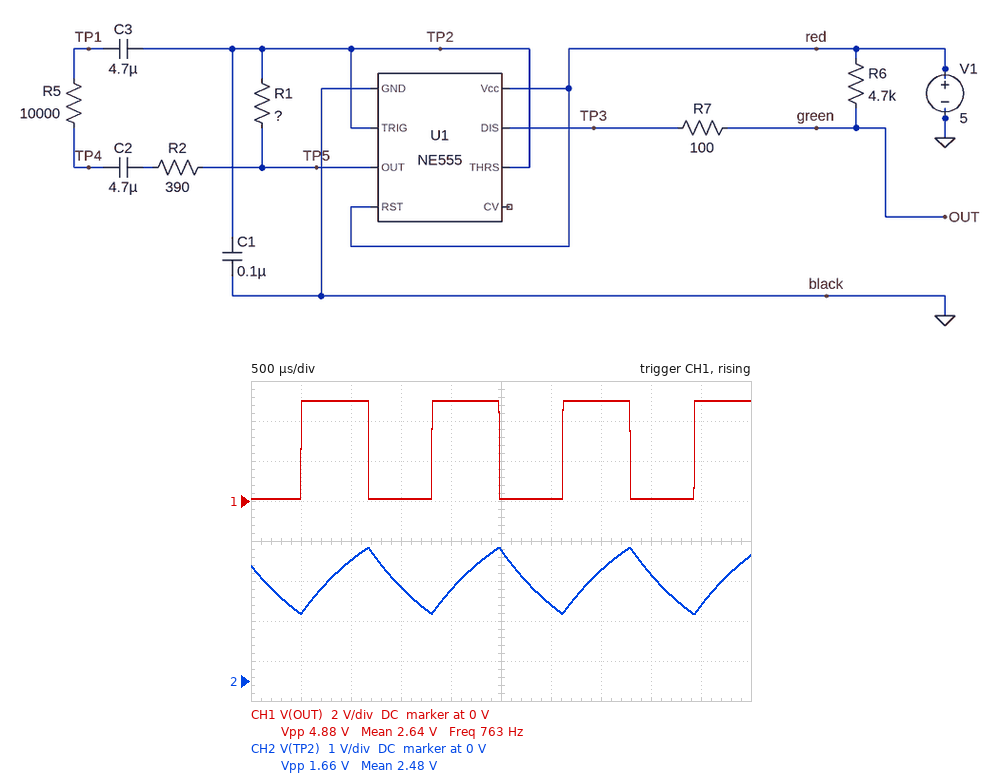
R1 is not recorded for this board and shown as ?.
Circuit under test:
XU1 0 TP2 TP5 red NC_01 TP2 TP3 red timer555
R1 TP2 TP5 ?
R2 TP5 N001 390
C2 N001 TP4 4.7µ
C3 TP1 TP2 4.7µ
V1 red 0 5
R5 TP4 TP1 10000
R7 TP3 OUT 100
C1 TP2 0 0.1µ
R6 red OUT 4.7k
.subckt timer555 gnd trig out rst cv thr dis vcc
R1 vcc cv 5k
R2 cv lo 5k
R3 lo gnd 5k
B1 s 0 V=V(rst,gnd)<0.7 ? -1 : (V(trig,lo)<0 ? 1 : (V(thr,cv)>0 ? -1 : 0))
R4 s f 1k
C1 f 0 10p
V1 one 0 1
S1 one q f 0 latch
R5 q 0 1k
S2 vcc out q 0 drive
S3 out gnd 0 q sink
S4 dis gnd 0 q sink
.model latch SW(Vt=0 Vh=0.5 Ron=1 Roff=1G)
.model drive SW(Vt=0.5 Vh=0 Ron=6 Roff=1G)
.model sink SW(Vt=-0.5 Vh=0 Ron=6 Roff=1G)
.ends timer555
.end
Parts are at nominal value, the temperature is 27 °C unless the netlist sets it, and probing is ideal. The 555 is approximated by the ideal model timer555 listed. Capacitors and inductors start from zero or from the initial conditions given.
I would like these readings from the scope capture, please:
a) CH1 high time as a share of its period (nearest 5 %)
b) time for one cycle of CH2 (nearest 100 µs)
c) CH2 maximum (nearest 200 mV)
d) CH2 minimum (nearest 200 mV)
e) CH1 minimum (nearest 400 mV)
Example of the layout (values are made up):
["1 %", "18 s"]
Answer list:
["50 %", "1.3 ms", "3.4 V", "1.6 V", "0 V"]
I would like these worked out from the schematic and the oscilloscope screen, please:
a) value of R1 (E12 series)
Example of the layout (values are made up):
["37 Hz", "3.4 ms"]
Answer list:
["100 kΩ"]
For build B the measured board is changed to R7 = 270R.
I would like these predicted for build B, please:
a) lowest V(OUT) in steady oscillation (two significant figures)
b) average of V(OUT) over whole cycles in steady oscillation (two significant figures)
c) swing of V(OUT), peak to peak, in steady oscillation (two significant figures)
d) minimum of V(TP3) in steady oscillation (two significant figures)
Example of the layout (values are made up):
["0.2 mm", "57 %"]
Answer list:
["280 mV", "2.7 V", "4.7 V", "6.0 mV"]
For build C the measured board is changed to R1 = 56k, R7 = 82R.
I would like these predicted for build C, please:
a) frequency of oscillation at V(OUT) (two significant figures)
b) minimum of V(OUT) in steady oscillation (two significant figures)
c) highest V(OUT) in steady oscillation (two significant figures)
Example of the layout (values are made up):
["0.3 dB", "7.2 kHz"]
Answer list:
["820 Hz", "92 mV", "5.0 V"]
